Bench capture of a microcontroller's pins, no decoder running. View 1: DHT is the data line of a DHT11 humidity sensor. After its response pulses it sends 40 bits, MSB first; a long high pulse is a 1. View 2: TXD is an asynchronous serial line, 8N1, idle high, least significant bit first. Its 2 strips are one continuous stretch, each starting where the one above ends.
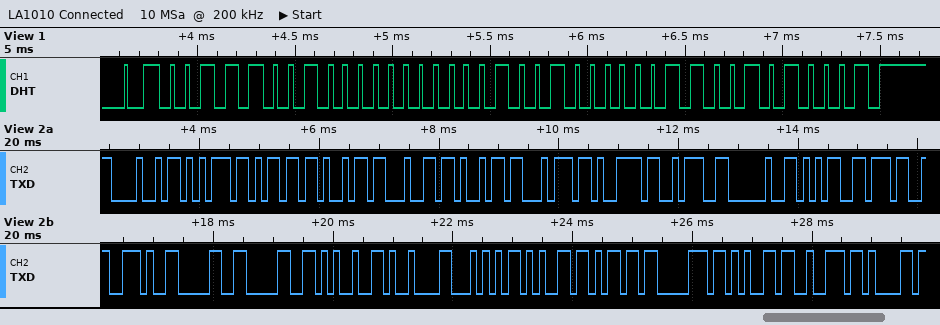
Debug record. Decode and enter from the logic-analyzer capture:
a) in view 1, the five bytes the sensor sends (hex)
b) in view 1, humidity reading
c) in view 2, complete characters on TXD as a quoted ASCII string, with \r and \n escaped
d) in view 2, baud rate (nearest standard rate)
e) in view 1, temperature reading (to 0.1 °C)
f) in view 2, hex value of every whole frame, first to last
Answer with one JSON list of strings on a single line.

["39 00 12 06 51", "57 %", "\"Humidity: 57.00%\\tTempera\"", "9600 baud", "18.6 °C", "48 75 6D 69 64 69 74 79 3A 20 35 37 2E 30 30 25 09 54 65 6D 70 65 72 61"]
